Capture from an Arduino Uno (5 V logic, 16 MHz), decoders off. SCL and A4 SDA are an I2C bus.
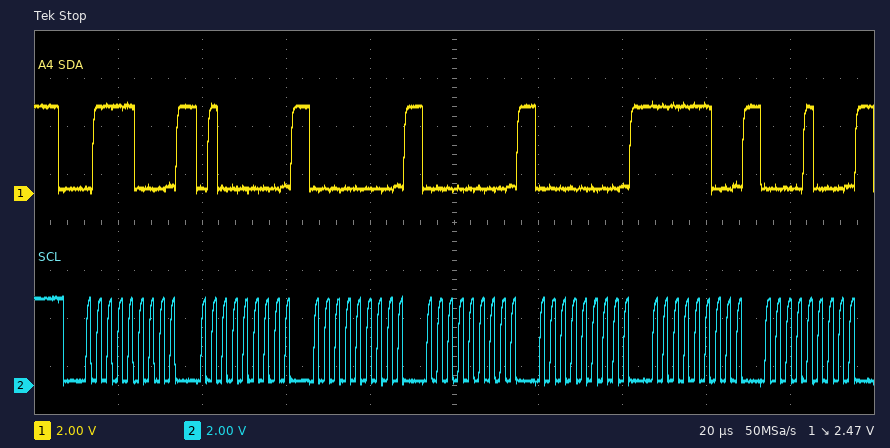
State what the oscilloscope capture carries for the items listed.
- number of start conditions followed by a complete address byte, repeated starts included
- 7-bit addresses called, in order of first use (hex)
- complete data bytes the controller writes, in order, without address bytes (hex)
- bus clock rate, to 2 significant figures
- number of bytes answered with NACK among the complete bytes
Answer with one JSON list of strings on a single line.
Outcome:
["1", "0x3C", "40 00 00 00 FC 08", "400 kHz", "0"]
